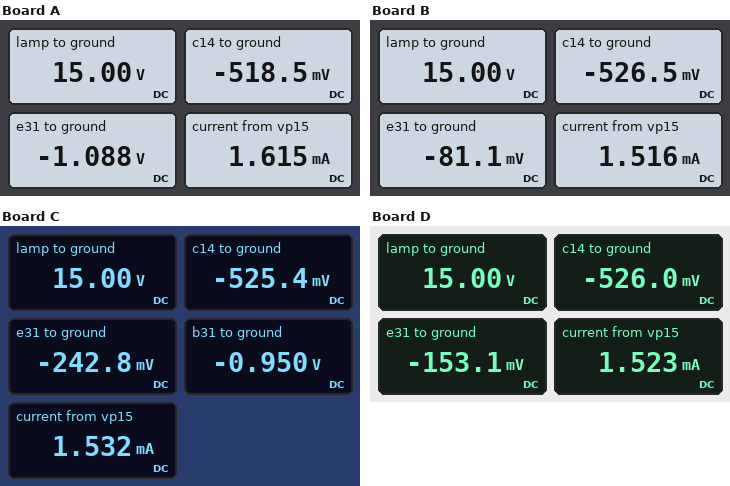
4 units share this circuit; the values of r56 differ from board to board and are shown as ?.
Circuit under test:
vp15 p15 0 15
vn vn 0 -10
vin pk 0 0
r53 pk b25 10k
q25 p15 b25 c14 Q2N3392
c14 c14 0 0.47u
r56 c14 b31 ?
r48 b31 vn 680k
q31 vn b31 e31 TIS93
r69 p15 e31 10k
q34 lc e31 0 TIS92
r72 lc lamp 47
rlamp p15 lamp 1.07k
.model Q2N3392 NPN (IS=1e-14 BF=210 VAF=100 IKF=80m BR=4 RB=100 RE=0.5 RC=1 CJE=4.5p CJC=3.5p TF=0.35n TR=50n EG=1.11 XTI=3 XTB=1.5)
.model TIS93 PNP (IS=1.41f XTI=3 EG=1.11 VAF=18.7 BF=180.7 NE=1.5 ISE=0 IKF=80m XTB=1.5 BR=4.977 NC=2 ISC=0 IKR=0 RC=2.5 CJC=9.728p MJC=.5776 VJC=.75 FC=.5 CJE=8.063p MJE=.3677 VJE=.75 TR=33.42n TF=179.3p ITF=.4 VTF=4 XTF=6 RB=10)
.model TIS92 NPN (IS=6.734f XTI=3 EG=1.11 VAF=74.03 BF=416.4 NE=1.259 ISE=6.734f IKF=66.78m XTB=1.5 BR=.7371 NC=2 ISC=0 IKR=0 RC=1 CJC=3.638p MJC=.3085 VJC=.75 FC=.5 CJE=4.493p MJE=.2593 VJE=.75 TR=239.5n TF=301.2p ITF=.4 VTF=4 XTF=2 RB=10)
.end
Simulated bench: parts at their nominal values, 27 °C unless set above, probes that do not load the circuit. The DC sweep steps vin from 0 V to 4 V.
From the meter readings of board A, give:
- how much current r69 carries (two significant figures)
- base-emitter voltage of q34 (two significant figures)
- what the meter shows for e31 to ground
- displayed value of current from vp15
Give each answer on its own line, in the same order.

1.6 mA
-1.1 V
-1.088 V
1.615 mA
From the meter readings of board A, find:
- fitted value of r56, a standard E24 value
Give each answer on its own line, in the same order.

220 kΩ
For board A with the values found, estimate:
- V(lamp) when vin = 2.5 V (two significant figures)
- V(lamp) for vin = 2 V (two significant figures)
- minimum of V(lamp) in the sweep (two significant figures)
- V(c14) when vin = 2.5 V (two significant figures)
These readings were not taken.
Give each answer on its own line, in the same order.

15 V
15 V
720 mV
2.0 V
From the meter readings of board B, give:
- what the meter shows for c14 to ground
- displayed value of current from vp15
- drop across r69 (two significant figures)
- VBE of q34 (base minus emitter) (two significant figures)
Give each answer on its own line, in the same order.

-526.5 mV
1.516 mA
15 V
-81 mV
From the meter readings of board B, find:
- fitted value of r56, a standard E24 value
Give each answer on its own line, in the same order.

33 kΩ
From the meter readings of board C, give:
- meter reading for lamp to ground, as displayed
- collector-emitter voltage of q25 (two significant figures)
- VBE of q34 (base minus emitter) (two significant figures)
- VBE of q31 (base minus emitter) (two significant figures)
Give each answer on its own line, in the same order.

15.00 V
16 V
-240 mV
-710 mV
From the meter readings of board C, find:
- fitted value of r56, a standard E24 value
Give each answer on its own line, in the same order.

56 kΩ
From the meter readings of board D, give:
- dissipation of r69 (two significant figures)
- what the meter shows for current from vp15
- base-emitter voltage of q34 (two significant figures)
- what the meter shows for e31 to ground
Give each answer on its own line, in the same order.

23 mW
1.523 mA
-150 mV
-153.1 mV
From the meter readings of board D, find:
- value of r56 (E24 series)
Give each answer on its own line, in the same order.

43 kΩ
